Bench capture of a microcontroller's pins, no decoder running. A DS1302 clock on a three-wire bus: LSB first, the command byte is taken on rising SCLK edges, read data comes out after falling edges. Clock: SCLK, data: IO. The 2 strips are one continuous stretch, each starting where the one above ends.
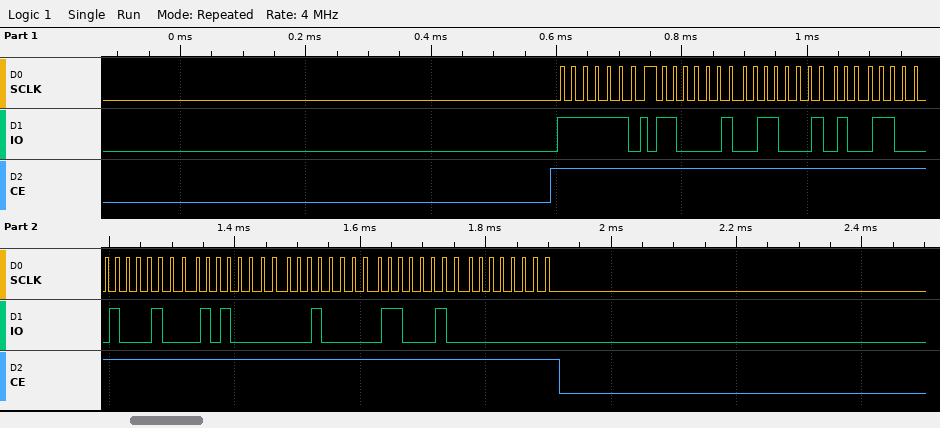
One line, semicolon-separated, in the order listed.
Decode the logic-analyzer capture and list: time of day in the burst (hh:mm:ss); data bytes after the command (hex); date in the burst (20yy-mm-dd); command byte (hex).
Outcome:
19:46:43; 43 46 19 11 05 04 23 00; 2023-05-11; 0xBF
